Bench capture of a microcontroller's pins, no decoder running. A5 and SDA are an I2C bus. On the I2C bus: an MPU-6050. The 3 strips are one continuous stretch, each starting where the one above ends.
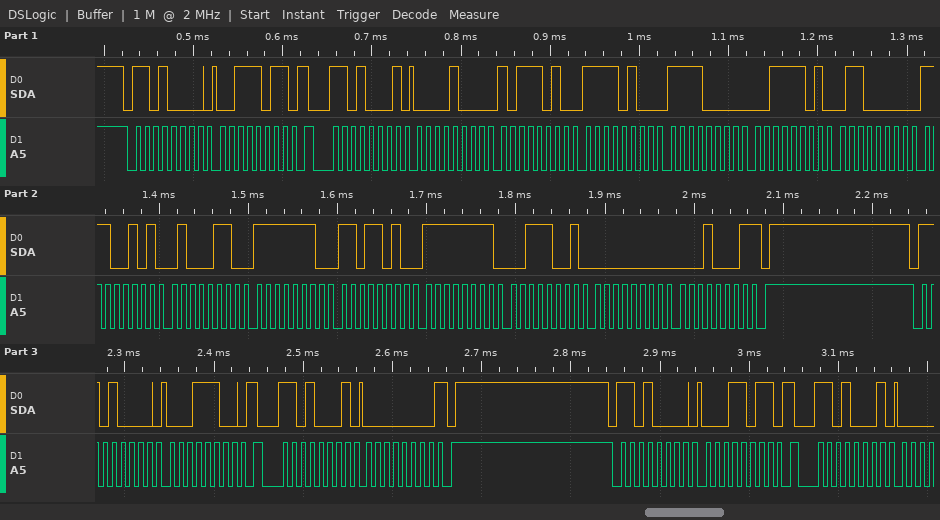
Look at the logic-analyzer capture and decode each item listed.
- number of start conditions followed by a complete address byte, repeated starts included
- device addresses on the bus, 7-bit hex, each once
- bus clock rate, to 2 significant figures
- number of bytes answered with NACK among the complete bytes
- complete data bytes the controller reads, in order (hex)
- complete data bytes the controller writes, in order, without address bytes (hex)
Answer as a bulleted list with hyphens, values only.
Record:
- 6
- 0x68
- 100 kHz
- 2
- 08 BA F4 F0 3D 60 E5 46 FE DA FF 39 00 11 00
- 3B 1C 1B
